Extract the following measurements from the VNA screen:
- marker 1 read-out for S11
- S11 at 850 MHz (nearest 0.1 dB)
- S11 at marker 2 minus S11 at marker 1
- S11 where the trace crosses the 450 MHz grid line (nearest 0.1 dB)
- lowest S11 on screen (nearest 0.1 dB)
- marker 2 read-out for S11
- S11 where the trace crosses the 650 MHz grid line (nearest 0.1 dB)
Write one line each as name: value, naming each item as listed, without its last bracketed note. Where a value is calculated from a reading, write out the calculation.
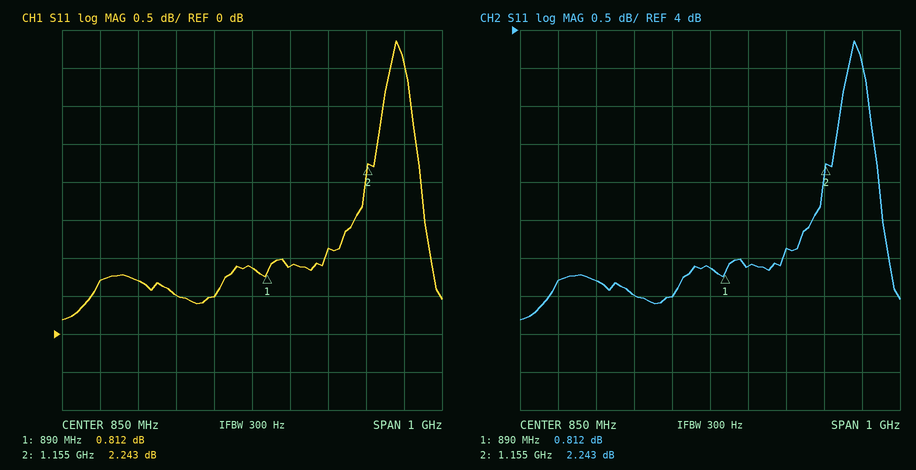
marker 1 read-out for S11: 0.812 dB
S11 at 850 MHz: 0.9 dB
S11 at marker 2 minus S11 at marker 1: 2.243 − (0.812) = 1.431 dB
S11 where the trace crosses the 450 MHz grid line: 0.7 dB
lowest S11 on screen: 0.2 dB
marker 2 read-out for S11: 2.243 dB
S11 where the trace crosses the 650 MHz grid line: 0.5 dB
